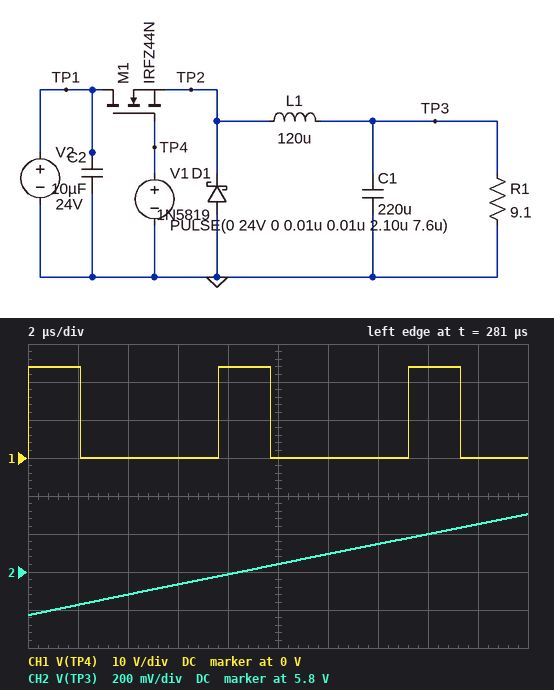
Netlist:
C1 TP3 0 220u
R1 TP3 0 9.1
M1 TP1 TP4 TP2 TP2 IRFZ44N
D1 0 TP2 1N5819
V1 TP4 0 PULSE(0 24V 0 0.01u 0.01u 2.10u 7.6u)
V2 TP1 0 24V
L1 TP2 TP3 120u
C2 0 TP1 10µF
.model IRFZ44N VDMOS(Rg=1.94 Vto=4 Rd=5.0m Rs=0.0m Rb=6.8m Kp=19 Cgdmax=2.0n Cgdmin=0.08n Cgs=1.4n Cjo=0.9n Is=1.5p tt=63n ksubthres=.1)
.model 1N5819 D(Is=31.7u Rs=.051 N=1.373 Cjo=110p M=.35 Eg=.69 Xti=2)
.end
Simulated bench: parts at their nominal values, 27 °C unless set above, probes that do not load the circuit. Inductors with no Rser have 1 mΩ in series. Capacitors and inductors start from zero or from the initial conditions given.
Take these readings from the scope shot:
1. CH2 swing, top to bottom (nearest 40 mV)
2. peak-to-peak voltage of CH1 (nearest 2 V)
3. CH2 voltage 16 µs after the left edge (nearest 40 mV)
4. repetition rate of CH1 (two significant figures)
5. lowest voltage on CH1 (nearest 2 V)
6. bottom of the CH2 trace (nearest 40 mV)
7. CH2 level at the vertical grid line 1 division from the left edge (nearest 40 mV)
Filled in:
520 mV
24 V
6.00 V
130 kHz
0 V
5.56 V
5.64 V
